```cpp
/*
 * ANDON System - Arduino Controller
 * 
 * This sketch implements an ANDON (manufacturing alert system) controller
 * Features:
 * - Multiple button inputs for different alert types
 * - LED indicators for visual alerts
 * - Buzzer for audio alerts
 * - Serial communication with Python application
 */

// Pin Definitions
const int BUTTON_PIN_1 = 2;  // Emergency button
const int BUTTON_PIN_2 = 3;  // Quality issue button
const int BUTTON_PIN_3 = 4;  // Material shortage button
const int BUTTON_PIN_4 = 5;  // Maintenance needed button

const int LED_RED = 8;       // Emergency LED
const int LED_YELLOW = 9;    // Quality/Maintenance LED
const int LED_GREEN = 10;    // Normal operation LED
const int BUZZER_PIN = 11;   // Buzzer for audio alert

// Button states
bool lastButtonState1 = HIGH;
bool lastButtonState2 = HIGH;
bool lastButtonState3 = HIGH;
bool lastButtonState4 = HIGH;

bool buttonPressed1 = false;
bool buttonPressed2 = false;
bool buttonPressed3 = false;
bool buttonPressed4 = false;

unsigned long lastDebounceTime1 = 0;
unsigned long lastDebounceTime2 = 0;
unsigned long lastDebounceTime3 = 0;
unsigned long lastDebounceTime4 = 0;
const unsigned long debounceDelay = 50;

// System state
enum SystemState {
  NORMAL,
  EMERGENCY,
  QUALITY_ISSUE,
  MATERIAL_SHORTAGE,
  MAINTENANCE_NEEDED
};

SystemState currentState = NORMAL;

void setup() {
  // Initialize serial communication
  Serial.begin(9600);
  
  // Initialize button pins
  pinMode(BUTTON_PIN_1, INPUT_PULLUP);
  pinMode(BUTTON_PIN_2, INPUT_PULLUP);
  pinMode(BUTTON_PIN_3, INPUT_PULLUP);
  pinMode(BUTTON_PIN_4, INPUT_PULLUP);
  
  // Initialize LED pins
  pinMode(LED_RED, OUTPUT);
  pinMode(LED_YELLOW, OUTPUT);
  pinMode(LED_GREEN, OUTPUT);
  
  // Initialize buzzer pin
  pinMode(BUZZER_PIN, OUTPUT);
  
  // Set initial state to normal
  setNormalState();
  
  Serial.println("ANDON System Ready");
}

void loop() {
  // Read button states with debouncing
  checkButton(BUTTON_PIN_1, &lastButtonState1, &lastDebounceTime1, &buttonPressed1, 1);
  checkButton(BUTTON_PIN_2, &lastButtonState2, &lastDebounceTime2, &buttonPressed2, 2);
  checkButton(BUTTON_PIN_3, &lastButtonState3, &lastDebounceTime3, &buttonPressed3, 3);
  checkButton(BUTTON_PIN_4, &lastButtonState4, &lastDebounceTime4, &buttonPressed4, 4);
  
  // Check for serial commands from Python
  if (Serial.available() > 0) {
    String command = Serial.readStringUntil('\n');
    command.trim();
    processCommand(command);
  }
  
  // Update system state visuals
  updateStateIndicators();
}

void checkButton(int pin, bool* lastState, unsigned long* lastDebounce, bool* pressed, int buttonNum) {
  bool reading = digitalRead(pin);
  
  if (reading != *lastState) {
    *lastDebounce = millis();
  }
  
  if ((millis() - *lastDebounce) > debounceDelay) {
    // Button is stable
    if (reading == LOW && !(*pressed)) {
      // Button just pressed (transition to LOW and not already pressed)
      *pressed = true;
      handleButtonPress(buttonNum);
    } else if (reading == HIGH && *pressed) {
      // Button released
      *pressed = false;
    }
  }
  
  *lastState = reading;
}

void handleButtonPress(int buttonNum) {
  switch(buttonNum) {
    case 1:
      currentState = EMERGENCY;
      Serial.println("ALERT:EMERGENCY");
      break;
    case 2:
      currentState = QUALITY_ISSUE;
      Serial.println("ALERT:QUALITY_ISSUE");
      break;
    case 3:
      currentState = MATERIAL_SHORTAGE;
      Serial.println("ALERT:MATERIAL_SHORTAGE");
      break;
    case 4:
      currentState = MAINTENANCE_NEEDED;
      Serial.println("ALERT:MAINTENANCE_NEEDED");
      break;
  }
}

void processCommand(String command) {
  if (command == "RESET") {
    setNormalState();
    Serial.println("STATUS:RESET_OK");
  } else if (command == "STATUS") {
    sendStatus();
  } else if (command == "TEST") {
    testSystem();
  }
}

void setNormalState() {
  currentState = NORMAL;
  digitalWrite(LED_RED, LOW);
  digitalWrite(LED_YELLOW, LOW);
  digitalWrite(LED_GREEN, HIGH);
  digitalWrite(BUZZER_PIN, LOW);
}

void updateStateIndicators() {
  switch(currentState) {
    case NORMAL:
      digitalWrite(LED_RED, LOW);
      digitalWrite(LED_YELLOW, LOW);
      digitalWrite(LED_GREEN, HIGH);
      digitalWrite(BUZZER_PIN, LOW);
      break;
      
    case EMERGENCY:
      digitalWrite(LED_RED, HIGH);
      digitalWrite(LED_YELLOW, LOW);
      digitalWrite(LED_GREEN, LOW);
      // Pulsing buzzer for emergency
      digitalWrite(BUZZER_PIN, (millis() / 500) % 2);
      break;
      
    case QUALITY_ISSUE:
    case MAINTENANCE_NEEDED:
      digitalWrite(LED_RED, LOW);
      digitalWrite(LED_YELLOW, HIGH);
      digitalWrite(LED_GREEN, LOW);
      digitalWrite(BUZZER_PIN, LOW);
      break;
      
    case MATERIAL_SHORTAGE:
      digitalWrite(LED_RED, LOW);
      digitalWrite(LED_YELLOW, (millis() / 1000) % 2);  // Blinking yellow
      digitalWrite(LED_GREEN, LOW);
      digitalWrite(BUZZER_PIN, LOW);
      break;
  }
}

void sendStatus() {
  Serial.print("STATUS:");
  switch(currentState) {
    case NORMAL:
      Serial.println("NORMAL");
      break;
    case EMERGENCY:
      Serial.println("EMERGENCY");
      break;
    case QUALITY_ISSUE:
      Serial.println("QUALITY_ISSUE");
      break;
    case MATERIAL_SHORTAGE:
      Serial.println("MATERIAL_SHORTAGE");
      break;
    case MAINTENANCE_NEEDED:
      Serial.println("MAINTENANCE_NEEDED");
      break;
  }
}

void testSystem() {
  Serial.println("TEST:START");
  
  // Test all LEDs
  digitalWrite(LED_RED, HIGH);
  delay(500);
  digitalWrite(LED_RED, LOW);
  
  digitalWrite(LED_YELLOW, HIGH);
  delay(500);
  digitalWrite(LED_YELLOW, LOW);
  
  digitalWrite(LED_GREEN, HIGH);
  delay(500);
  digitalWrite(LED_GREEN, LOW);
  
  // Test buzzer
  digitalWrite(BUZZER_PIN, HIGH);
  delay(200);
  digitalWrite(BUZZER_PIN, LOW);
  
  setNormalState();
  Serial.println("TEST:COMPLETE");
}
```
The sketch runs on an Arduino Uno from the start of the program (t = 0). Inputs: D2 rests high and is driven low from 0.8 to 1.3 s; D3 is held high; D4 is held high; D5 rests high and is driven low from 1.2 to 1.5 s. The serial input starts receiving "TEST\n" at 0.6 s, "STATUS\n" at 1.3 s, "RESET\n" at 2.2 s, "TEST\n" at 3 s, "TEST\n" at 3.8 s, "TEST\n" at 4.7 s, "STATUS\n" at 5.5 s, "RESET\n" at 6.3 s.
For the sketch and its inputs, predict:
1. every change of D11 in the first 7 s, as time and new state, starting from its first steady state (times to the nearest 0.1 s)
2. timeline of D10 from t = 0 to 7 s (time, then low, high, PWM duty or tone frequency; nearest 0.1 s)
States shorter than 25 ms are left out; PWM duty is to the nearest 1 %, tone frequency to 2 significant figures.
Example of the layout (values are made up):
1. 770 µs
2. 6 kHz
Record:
1. 0 s low; 2.1 s high; 2.3 s low; 4.5 s high; 4.7 s low; 6.2 s high; 6.4 s low
2. 0 s high; 2.1 s low; 2.3 s high; 4.5 s low; 4.7 s high; 6.2 s low; 6.4 s high
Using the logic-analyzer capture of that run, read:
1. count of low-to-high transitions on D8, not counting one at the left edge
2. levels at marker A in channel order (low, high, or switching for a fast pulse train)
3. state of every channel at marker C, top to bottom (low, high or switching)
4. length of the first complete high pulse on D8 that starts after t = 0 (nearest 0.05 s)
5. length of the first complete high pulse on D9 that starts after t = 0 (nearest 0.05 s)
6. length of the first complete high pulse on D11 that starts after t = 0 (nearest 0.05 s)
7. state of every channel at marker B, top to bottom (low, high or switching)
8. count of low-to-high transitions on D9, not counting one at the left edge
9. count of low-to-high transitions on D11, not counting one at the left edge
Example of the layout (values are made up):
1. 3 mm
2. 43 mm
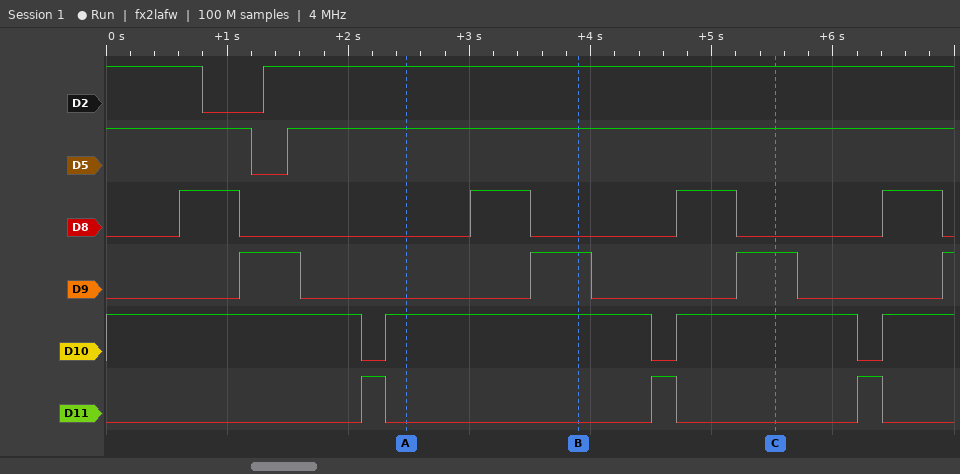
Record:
1. 4
2. D2 high, D5 high, D8 low, D9 low, D10 high, D11 low
3. D2 high, D5 high, D8 low, D9 high, D10 high, D11 low
4. 0.50 s
5. 0.50 s
6. 0.20 s
7. D2 high, D5 high, D8 low, D9 high, D10 high, D11 low
8. 4
9. 3
